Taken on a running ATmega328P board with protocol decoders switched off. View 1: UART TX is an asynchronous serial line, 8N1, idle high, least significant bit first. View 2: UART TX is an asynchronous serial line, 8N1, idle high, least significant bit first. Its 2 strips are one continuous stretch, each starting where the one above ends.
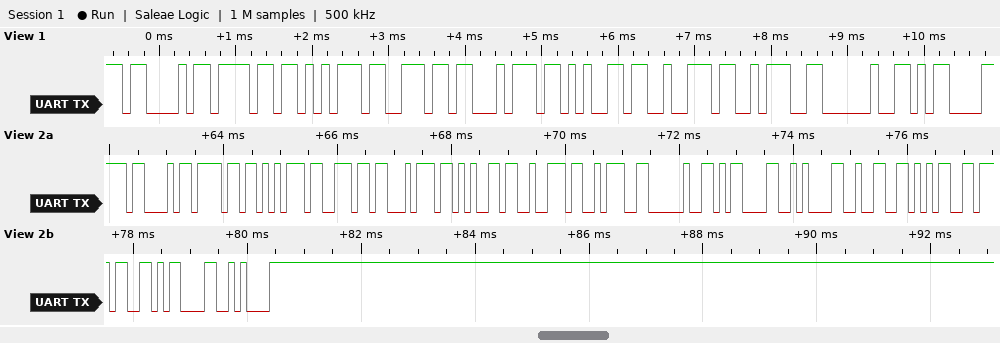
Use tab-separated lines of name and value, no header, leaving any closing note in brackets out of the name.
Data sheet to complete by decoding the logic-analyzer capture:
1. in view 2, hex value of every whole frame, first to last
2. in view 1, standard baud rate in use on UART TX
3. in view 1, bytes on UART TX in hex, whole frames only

in view 2, hex value of every whole frame, first to last	0x43 0x6F 0x75 0x6E 0x74 0x65 0x72 0x3A 0x20 0x0D 0x0A 0x32 0x35 0x37 0x0D 0x0A
in view 1, standard baud rate in use on UART TX	9600 baud
in view 1, bytes on UART TX in hex, whole frames only	43 6F 75 6E 74 65 72 3A 20 0D
